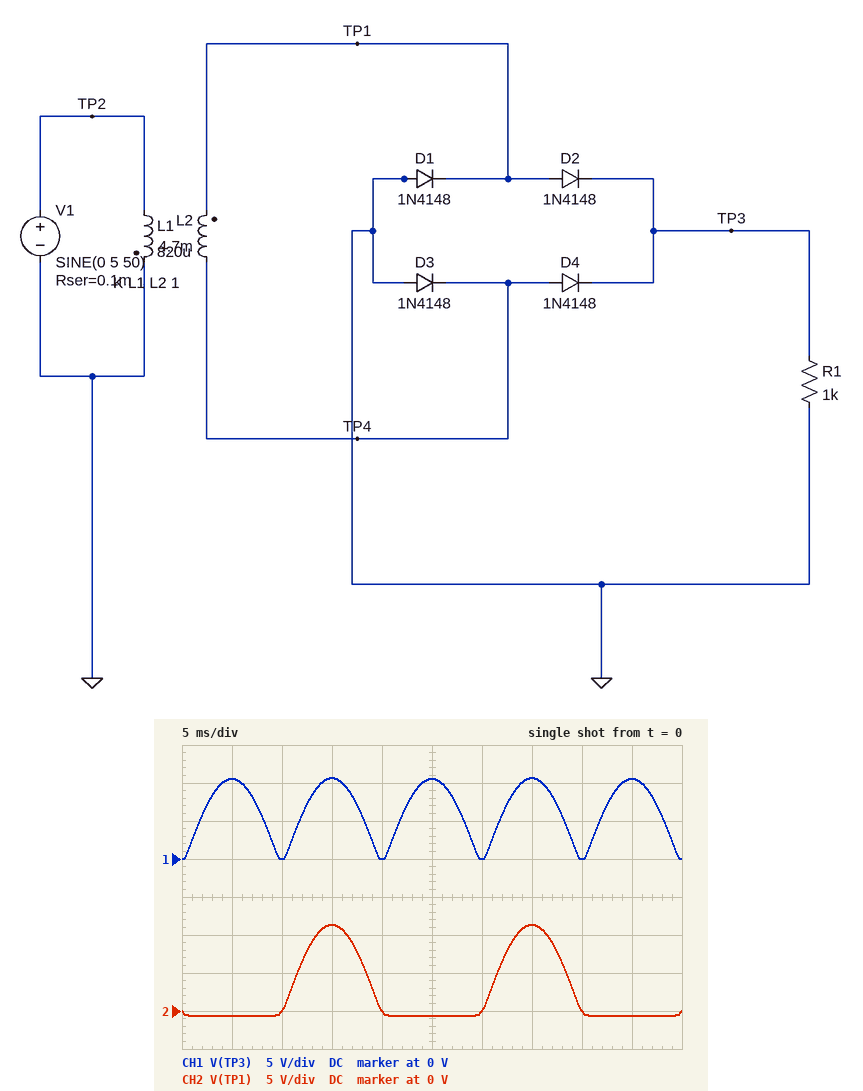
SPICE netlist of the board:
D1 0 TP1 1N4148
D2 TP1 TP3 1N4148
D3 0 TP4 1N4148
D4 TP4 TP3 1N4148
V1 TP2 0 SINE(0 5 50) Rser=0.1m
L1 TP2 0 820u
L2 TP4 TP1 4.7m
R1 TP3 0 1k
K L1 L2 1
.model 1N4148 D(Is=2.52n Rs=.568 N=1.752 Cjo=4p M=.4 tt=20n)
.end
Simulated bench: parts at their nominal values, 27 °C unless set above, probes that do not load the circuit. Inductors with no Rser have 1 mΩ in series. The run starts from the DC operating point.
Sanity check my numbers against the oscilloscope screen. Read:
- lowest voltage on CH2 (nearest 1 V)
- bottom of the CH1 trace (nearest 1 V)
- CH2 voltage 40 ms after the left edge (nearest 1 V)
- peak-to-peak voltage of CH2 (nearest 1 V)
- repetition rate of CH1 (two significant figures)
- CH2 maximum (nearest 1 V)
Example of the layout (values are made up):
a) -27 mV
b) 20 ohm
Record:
a) -1 V
b) 0 V
c) 0 V
d) 12 V
e) 100 Hz
f) 11 V
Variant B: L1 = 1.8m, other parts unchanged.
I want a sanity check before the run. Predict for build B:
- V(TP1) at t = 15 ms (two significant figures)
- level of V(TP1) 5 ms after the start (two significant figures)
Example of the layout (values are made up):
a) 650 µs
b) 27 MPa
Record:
a) 7.4 V
b) -670 mV
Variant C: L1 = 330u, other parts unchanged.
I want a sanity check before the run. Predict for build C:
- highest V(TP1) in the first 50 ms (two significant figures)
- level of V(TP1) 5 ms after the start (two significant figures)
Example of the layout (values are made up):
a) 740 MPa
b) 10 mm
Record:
a) 18 V
b) -720 mV
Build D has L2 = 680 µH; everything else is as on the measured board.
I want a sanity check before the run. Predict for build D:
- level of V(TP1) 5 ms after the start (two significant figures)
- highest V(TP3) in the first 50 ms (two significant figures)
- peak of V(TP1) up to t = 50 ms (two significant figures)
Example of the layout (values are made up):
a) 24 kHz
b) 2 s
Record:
a) -640 mV
b) 3.3 V
c) 3.9 V
